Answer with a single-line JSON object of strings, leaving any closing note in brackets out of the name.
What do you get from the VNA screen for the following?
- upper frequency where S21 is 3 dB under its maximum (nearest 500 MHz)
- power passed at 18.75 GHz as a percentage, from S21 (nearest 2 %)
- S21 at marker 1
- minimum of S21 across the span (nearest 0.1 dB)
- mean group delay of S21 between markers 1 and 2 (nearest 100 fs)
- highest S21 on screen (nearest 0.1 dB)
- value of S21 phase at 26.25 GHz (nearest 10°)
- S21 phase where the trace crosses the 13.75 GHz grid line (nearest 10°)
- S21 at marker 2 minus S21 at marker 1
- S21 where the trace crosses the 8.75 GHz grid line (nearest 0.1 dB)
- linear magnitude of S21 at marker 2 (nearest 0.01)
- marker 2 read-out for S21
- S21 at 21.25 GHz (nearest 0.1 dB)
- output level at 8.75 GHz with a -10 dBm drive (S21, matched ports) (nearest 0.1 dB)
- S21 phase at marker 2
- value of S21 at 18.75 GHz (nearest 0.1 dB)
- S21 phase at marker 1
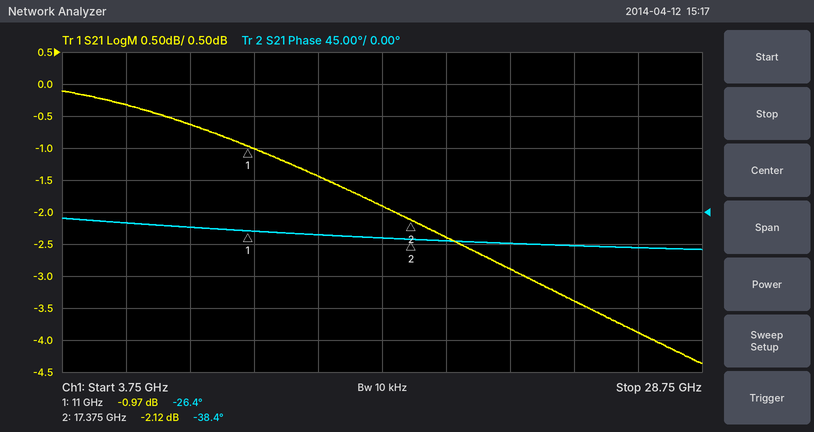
{"upper frequency where S21 is 3 dB under its maximum": "22.5 GHz", "power passed at 18.75 GHz as a percentage, from S21": "58 %", "S21 at marker 1": "-0.97 dB", "minimum of S21 across the span": "-4.4 dB", "mean group delay of S21 between markers 1 and 2": "5.2 ps", "highest S21 on screen": "-0.1 dB", "value of S21 phase at 26.25 GHz": "-50°", "S21 phase where the trace crosses the 13.75 GHz grid line": "-30°", "S21 at marker 2 minus S21 at marker 1": "-1.15 dB", "S21 where the trace crosses the 8.75 GHz grid line": "-0.6 dB", "linear magnitude of S21 at marker 2": "0.78", "marker 2 read-out for S21": "-2.12 dB", "S21 at 21.25 GHz": "-2.9 dB", "output level at 8.75 GHz with a -10 dBm drive (S21, matched ports)": "-10.6 dBm", "S21 phase at marker 2": "-38.4°", "value of S21 at 18.75 GHz": "-2.4 dB", "S21 phase at marker 1": "-26.4°"}
